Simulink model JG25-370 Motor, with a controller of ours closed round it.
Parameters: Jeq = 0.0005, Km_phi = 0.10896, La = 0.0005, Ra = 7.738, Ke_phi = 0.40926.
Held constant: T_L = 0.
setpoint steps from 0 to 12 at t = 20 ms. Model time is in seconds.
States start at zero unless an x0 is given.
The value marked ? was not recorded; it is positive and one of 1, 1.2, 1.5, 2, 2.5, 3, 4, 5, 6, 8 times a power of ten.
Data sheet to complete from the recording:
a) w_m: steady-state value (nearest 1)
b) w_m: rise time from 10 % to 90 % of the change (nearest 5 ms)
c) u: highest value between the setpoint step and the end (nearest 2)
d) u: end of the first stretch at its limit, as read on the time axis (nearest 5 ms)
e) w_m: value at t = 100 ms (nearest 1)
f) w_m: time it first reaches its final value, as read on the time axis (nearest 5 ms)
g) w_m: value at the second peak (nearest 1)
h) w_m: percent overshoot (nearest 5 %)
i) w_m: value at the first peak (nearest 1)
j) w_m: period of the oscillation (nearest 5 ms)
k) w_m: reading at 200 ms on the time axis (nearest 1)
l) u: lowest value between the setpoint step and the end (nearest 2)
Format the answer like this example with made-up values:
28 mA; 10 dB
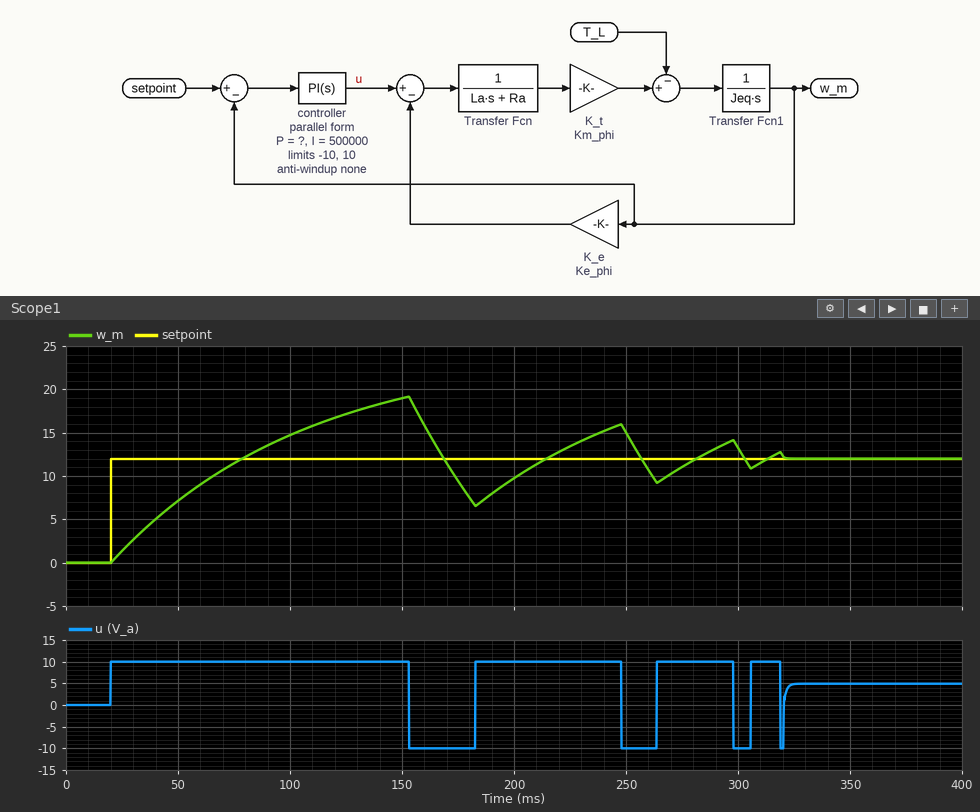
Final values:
12; 45 ms; 10; 155 ms; 15; 80 ms; 16; 60 %; 19; 95 ms; 10; -10
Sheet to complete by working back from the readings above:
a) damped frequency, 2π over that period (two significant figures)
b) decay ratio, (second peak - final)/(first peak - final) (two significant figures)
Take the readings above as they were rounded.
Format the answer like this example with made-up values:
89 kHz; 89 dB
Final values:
0.066 rad/ms; 0.57
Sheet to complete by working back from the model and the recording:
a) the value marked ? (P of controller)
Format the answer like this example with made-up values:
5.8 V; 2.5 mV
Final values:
600
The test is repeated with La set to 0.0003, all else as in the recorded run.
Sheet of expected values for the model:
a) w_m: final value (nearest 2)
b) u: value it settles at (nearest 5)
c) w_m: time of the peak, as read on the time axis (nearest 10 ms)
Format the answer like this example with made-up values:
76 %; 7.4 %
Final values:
12; 5; 150 ms
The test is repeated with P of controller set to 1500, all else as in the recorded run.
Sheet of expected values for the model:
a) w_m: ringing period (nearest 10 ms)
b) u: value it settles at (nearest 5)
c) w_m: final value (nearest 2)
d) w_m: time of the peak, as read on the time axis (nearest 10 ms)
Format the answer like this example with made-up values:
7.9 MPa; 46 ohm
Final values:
70 ms; 5; 12; 150 ms
